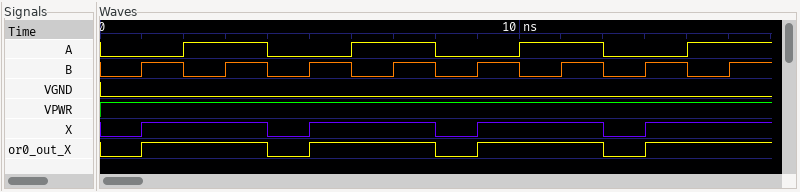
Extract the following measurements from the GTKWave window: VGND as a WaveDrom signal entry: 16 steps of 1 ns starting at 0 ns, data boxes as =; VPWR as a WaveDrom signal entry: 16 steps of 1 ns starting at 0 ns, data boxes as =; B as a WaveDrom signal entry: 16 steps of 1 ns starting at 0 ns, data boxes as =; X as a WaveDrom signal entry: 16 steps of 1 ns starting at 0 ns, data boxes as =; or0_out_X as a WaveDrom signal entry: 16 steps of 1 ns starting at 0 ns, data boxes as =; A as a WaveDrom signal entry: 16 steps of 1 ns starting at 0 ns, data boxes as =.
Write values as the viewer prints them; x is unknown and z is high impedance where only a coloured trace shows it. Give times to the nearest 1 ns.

{name: 'VGND', wave: '0...............'}
{name: 'VPWR', wave: '1...............'}
{name: 'B', wave: '0101010101010101'}
{name: 'X', wave: '01..01..01..01..'}
{name: 'or0_out_X', wave: '01..01..01..01..'}
{name: 'A', wave: '0.1.0.1.0.1.0.1.'}
